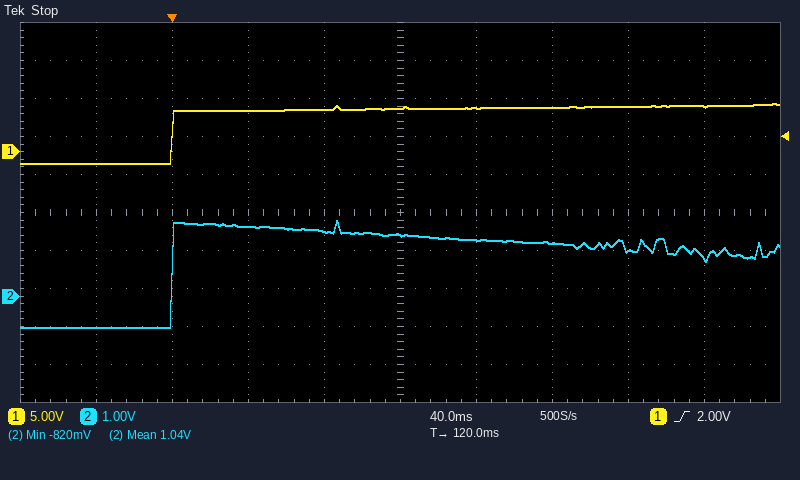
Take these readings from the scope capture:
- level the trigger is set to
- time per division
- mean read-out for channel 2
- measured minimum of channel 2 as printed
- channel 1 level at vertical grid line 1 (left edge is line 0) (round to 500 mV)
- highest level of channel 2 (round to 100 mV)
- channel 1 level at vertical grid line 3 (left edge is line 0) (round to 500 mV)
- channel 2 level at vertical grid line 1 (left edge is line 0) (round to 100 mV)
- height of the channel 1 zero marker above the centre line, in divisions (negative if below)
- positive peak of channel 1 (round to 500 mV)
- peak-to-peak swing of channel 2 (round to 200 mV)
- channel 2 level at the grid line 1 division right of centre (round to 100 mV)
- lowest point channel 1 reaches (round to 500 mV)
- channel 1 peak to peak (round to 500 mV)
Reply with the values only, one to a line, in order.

2.00 V
40 ms
1.04 V
-820 mV
-1.5 V
2.0 V
5.5 V
-800 mV
+1.6 div
6.5 V
2.8 V
1.5 V
-1.5 V
8.0 V
